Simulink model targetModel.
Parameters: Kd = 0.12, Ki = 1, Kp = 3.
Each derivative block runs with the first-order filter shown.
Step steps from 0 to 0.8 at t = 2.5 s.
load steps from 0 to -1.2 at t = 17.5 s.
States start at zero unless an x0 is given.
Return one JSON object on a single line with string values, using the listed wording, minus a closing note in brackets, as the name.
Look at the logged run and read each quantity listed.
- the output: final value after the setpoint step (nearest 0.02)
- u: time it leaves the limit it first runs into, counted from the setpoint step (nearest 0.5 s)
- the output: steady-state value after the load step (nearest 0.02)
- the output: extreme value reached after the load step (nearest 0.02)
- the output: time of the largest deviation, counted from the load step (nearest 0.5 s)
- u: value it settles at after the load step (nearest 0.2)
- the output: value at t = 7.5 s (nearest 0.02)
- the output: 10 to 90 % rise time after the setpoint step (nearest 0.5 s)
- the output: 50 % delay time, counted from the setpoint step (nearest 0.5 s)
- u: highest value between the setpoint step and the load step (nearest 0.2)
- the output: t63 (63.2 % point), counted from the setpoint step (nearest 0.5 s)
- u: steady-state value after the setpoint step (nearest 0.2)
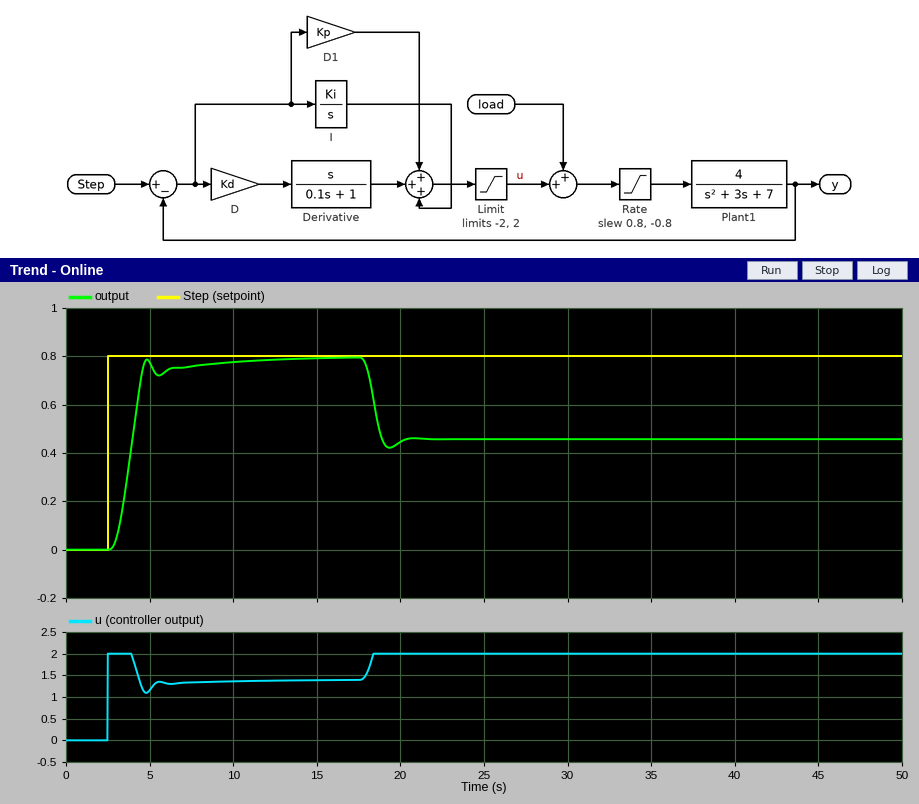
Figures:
{"the output: final value after the setpoint step": "0.80", "u: time it leaves the limit it first runs into, counted from the setpoint step": "1.5 s", "the output: steady-state value after the load step": "0.46", "the output: extreme value reached after the load step": "0.42", "the output: time of the largest deviation, counted from the load step": "2.0 s", "u: value it settles at after the load step": "2.0", "the output: value at t = 7.5 s": "0.76", "the output: 10 to 90 % rise time after the setpoint step": "1.5 s", "the output: 50 % delay time, counted from the setpoint step": "1.5 s", "u: highest value between the setpoint step and the load step": "2.0", "the output: t63 (63.2 % point), counted from the setpoint step": "1.5 s", "u: steady-state value after the setpoint step": "1.4"}
